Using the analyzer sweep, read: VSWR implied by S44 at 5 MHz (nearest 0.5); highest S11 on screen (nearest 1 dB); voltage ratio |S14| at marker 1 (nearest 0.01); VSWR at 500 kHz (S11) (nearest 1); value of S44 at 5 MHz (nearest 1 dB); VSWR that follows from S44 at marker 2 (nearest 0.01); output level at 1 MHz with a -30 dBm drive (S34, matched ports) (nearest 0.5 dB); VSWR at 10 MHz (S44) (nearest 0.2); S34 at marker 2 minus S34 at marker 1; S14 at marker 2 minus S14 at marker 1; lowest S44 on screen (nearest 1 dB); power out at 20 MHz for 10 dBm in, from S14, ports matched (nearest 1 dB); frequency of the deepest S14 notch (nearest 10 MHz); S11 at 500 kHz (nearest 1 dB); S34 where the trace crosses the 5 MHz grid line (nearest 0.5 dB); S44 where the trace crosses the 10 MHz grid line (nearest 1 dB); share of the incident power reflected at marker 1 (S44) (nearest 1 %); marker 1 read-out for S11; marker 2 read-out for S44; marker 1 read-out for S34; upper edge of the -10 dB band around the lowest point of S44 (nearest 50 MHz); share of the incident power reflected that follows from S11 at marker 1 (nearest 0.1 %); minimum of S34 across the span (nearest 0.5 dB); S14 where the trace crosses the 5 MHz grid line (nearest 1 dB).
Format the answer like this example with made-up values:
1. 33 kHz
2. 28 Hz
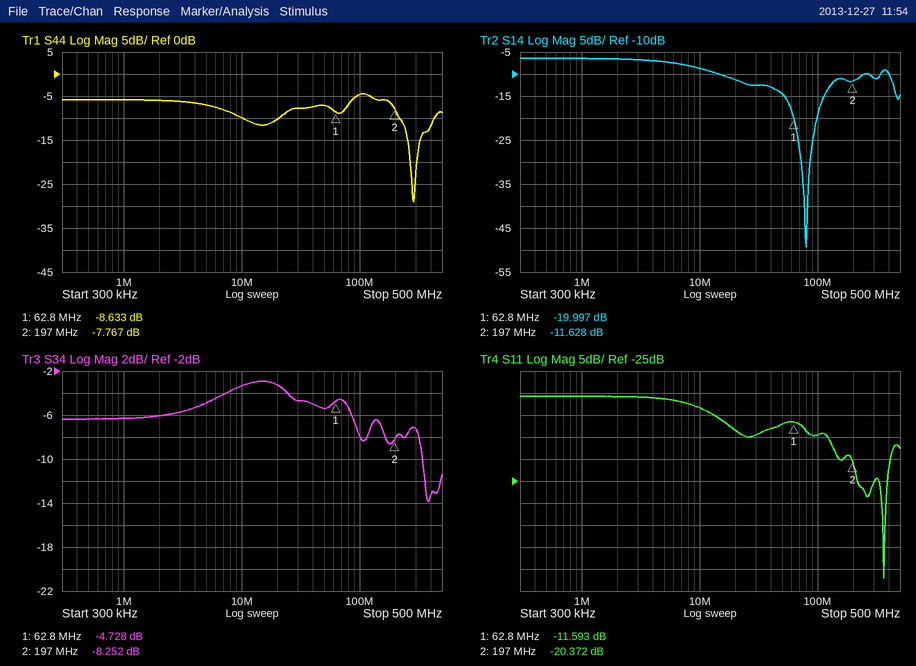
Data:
1. 2.5
2. -6 dB
3. 0.10
4. 3
5. -7 dB
6. 2.38
7. -36.5 dBm
8. 2.0
9. -3.524 dB
10. 8.369 dB
11. -29 dB
12. -1 dBm
13. 80 MHz
14. -6 dB
15. -5.0 dB
16. -10 dB
17. 14 %
18. -11.593 dB
19. -7.767 dB
20. -4.728 dB
21. 450 MHz
22. 6.9 %
23. -14.0 dB
24. -7 dB
